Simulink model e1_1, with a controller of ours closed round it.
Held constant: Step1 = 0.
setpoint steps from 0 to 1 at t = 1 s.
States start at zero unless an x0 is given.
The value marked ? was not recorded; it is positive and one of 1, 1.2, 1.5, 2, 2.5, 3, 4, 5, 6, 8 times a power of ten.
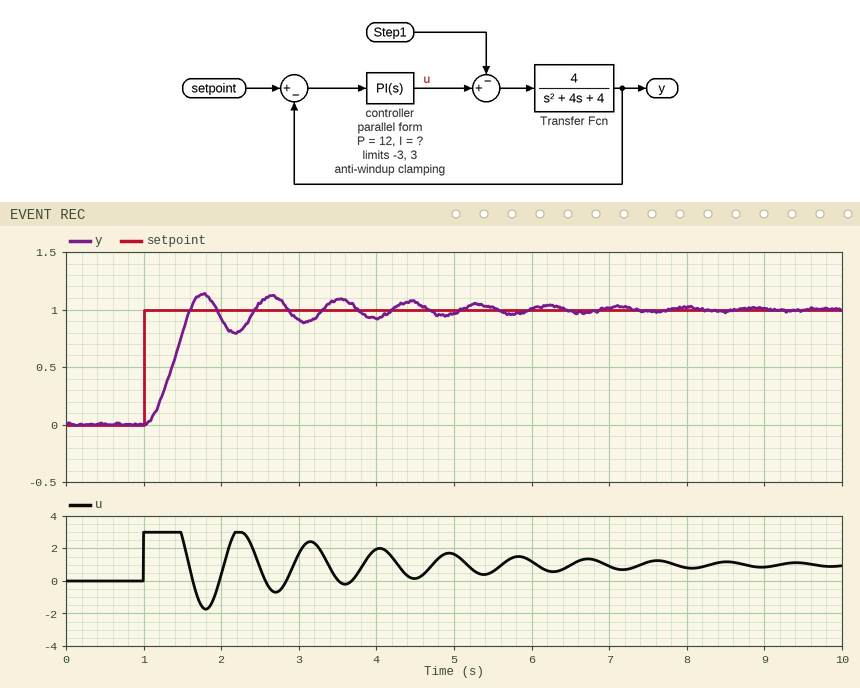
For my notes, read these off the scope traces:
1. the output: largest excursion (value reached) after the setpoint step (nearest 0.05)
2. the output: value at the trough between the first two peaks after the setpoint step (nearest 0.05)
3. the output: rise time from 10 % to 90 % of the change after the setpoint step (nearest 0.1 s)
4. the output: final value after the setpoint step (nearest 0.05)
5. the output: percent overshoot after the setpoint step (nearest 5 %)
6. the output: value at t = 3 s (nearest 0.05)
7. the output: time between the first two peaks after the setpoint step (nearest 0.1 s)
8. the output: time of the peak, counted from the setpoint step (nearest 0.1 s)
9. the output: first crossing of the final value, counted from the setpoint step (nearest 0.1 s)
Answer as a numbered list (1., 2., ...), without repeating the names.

1. 1.15
2. 0.80
3. 0.4 s
4. 1.00
5. 15 %
6. 0.90
7. 0.9 s
8. 0.8 s
9. 0.6 s
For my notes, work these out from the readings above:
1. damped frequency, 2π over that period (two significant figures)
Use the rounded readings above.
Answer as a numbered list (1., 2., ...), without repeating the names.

1. 7.0 rad/s
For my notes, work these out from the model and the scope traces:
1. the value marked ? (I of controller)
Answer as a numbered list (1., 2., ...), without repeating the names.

1. 40
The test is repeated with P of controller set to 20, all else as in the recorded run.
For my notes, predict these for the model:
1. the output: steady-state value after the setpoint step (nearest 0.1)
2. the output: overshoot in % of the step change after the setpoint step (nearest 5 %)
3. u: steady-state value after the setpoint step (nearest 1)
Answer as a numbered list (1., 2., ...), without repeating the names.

1. 1.0
2. 10 %
3. 1
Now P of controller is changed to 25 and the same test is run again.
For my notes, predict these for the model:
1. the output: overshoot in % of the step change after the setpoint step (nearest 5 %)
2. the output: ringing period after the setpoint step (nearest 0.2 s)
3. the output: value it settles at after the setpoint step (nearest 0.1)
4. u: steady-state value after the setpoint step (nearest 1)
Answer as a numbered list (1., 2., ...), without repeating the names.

1. 10 %
2. 0.6 s
3. 1.0
4. 1
